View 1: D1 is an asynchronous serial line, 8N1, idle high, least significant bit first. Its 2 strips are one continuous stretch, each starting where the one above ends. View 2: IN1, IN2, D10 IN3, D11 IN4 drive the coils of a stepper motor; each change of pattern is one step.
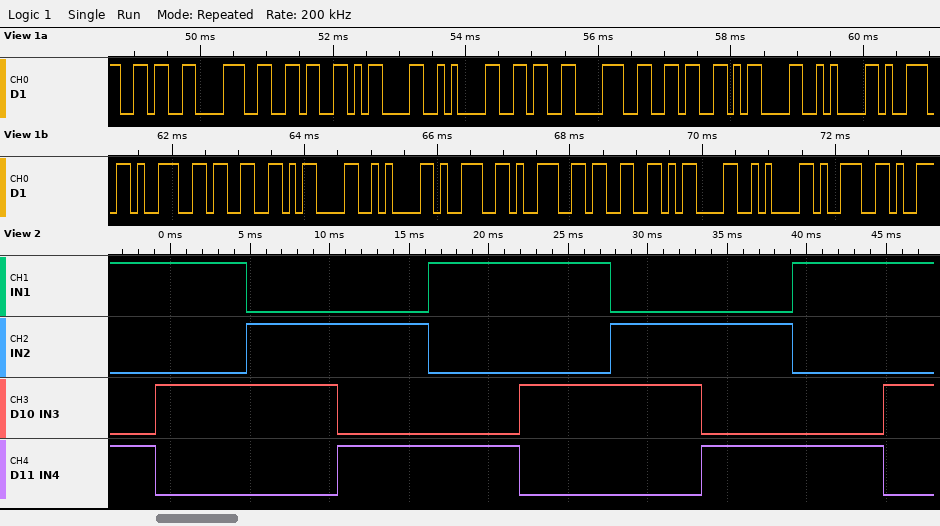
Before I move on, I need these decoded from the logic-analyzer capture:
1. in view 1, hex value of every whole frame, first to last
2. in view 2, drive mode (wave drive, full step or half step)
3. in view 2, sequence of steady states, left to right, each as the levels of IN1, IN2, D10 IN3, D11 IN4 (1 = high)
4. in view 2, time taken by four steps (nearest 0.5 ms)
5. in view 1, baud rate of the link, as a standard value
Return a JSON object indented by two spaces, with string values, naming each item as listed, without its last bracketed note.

{
  "in view 1, hex value of every whole frame, first to last": "36 38 36 0D 0A 36 38 36 0D 0A 39 39 33 0D 0A 39 39 33 0D 0A 39",
  "in view 2, drive mode": "full step",
  "in view 2, sequence of steady states, left to right, each as the levels of IN1, IN2, D10 IN3, D11 IN4": "1001 1010 0110 0101 1001 1010 0110 0101 1001 1010",
  "in view 2, time taken by four steps": "23.0 ms",
  "in view 1, baud rate of the link, as a standard value": "9600 baud"
}
